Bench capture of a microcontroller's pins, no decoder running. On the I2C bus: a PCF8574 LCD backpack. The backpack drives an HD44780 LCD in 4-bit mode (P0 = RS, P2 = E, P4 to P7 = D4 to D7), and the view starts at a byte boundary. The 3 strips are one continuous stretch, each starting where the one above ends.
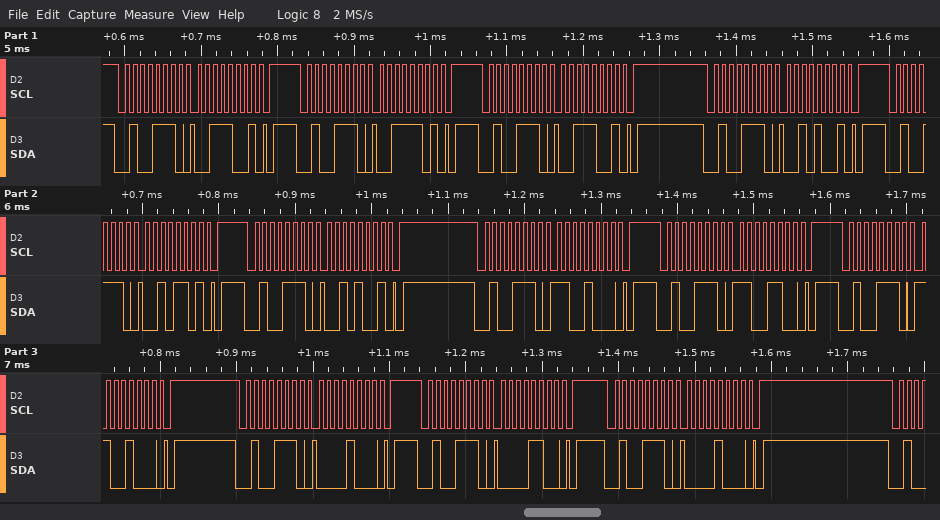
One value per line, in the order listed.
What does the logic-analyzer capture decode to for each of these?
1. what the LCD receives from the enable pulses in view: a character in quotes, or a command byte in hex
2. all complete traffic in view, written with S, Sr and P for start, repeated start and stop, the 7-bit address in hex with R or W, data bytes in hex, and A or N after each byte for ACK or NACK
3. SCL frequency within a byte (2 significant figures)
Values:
'2' 0xC0
S 27W A 39 A P S 27W A 3D A P S 27W A 39 A P S 27W A 29 A P S 27W A 2D A P S 27W A 29 A P S 27W A C8 A P S 27W A CC A P S 27W A C8 A P S 27W A 08 A P S 27W A 0C A P S 27W A 08 A P
100 kHz
